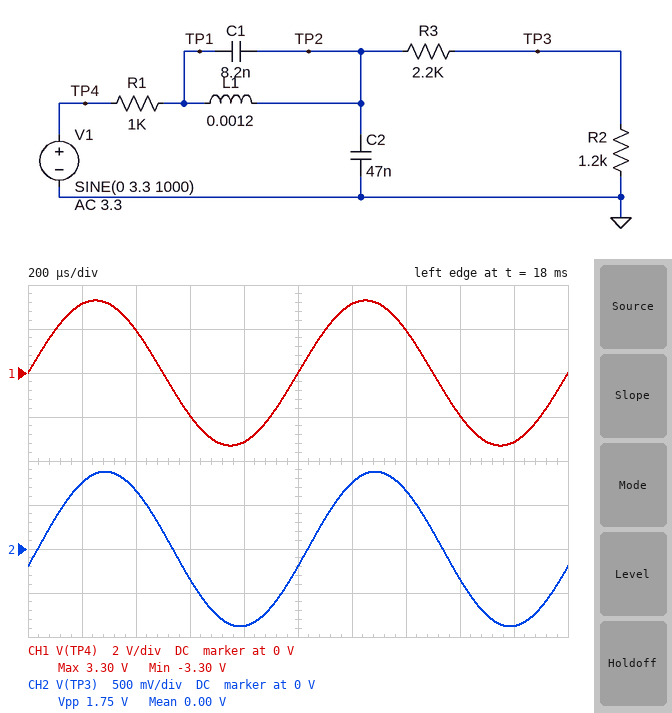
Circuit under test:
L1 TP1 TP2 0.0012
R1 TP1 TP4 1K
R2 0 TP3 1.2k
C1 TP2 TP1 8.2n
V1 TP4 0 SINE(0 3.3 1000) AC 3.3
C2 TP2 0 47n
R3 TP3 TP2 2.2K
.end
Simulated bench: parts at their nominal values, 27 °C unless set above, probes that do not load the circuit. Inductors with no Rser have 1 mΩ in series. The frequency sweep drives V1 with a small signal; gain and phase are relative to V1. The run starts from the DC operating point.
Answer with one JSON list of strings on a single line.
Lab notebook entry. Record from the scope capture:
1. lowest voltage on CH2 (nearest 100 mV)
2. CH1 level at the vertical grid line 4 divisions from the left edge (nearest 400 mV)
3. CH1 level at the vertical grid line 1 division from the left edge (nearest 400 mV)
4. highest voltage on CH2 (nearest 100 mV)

["-900 mV", "-3.2 V", "3.2 V", "900 mV"]
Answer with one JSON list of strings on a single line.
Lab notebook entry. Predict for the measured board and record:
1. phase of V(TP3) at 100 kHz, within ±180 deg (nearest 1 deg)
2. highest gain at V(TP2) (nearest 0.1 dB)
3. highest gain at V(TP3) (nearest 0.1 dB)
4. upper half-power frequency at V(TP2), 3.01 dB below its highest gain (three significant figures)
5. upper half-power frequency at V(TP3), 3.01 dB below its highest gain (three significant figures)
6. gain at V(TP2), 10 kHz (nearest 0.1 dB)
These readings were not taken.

["-73 deg", "-2.2 dB", "-11.3 dB", "4.50 kHz", "4.50 kHz", "-10.0 dB"]
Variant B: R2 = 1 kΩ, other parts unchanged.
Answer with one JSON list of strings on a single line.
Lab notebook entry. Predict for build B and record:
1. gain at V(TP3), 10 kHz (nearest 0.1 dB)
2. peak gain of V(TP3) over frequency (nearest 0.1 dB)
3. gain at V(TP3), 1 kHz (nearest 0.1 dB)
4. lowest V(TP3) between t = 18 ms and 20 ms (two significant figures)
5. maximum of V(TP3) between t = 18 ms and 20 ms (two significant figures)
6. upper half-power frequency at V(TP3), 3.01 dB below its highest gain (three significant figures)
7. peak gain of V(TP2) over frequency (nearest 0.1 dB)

["-20.1 dB", "-12.5 dB", "-12.7 dB", "-770 mV", "770 mV", "4.56 kHz", "-2.4 dB"]
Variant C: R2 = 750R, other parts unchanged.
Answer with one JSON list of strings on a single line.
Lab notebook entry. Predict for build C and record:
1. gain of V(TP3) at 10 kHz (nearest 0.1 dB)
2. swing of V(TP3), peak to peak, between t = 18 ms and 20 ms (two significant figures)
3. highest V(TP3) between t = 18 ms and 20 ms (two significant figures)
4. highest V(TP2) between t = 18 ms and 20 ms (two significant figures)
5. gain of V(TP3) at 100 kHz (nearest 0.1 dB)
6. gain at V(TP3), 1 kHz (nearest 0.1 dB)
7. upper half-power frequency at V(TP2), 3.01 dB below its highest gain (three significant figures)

["-21.9 dB", "1.2 V", "610 mV", "2.4 V", "-41.7 dB", "-14.6 dB", "4.65 kHz"]
